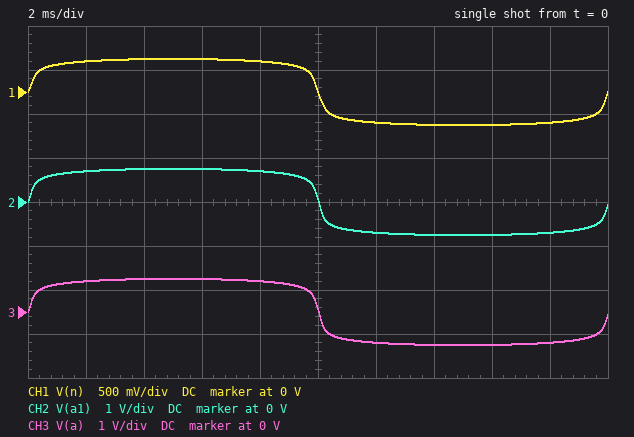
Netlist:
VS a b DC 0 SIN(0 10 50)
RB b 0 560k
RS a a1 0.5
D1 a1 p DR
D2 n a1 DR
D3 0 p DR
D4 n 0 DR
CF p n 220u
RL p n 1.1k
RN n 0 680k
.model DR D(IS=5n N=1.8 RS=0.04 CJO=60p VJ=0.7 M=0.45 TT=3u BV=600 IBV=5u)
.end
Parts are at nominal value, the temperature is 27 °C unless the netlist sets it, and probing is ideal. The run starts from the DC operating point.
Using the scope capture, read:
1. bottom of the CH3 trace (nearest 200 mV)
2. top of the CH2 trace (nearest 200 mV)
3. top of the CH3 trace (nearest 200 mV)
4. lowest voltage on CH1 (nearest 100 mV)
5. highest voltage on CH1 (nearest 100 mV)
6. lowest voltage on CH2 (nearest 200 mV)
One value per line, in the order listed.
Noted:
-800 mV
800 mV
800 mV
-400 mV
400 mV
-800 mV
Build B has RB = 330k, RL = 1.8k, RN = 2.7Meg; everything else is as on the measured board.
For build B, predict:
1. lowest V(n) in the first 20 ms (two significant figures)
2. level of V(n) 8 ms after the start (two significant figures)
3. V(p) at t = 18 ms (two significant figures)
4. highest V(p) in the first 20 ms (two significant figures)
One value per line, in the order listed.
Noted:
-400 mV
370 mV
-370 mV
400 mV
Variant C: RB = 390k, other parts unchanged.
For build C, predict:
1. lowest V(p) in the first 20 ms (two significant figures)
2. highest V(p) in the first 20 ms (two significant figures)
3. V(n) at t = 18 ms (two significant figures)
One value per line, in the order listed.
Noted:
-390 mV
390 mV
-370 mV
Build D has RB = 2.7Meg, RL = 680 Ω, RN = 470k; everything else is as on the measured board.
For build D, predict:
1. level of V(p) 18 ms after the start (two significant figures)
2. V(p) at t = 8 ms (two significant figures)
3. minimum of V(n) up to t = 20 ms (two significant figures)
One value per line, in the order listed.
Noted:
-260 mV
260 mV
-300 mV
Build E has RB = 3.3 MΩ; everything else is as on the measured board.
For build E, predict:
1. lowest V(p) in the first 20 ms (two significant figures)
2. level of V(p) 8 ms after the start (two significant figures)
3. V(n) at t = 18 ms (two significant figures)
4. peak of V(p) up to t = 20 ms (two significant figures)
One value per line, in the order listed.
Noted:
-290 mV
260 mV
-260 mV
290 mV
